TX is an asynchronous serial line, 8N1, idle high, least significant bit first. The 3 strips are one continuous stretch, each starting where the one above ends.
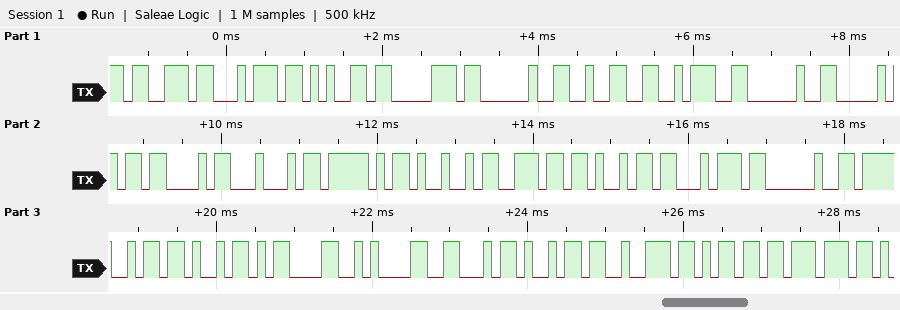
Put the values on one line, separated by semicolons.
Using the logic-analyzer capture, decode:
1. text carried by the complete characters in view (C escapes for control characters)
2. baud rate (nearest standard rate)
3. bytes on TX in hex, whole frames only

"step 2: PCD_Init OK\r\nFirmw"; 9600 baud; 73 74 65 70 20 32 3A 20 50 43 44 5F 49 6E 69 74 20 4F 4B 0D 0A 46 69 72 6D 77
